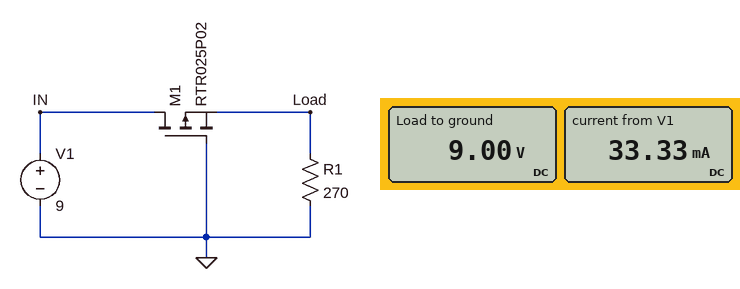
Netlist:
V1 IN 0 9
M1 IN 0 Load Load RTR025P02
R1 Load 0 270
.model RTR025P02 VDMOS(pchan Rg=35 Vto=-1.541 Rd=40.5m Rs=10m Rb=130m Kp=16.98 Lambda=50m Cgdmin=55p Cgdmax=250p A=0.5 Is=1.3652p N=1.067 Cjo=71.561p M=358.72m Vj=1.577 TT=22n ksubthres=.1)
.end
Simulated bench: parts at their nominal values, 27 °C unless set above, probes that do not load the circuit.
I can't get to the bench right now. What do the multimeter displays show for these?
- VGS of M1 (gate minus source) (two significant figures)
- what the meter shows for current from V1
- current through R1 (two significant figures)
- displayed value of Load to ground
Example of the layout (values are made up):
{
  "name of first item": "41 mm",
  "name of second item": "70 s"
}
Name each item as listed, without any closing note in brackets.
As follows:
{
  "VGS of M1 (gate minus source)": "-9.0 V",
  "what the meter shows for current from V1": "33.33 mA",
  "current through R1": "33 mA",
  "displayed value of Load to ground": "9.00 V"
}
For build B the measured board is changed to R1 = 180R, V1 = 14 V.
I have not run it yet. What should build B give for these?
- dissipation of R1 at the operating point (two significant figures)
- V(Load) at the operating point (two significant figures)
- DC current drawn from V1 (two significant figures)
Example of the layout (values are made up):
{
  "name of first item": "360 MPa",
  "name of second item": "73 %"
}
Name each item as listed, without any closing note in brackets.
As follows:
{
  "dissipation of R1 at the operating point": "1.1 W",
  "V(Load) at the operating point": "14 V",
  "DC current drawn from V1": "78 mA"
}
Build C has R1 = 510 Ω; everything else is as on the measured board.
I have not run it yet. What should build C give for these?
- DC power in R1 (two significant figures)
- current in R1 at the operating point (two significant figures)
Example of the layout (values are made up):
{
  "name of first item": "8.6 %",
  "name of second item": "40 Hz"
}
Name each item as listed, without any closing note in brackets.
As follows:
{
  "DC power in R1": "160 mW",
  "current in R1 at the operating point": "18 mA"
}
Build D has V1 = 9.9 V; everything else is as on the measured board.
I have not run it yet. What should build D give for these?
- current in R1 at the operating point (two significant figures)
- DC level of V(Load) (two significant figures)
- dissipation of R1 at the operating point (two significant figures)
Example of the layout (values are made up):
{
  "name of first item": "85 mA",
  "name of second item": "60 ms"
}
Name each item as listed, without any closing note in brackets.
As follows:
{
  "current in R1 at the operating point": "37 mA",
  "DC level of V(Load)": "9.9 V",
  "dissipation of R1 at the operating point": "360 mW"
}
